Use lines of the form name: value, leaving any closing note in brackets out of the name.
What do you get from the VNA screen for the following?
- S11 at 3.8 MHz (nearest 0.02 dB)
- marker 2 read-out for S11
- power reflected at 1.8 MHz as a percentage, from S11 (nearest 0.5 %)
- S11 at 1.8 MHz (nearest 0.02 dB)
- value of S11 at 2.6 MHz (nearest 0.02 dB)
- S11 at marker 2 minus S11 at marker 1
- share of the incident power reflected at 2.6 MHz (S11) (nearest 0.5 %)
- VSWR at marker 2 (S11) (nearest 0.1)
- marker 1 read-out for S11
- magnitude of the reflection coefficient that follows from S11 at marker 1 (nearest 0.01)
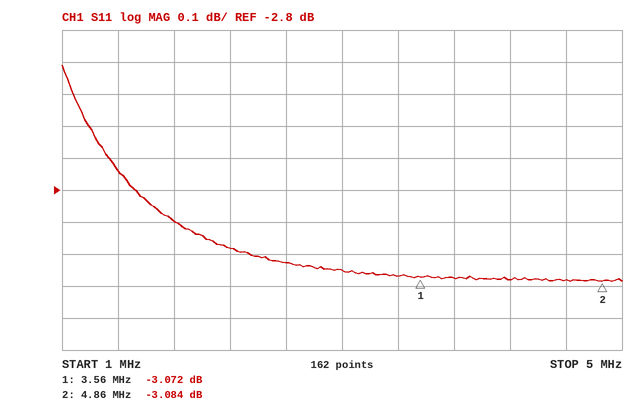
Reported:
S11 at 3.8 MHz: -3.08 dB
marker 2 read-out for S11: -3.084 dB
power reflected at 1.8 MHz as a percentage, from S11: 51.5 %
S11 at 1.8 MHz: -2.90 dB
value of S11 at 2.6 MHz: -3.02 dB
S11 at marker 2 minus S11 at marker 1: -0.012 dB
share of the incident power reflected at 2.6 MHz (S11): 50.0 %
VSWR at marker 2 (S11): 5.7
marker 1 read-out for S11: -3.072 dB
magnitude of the reflection coefficient that follows from S11 at marker 1: 0.70
